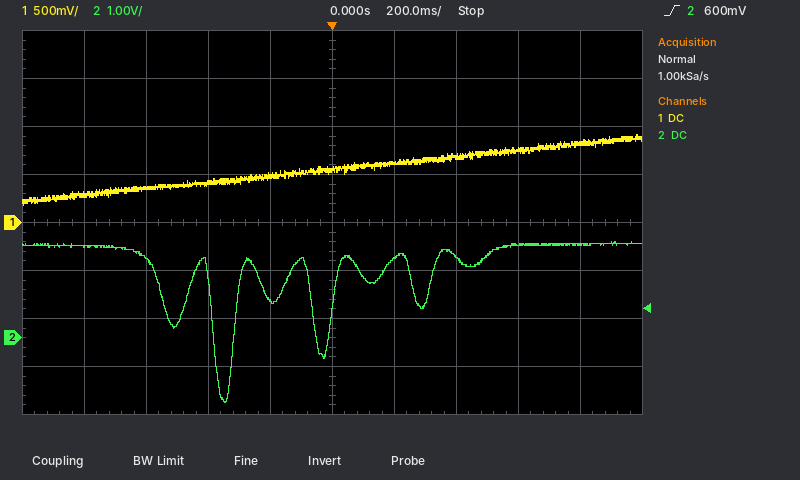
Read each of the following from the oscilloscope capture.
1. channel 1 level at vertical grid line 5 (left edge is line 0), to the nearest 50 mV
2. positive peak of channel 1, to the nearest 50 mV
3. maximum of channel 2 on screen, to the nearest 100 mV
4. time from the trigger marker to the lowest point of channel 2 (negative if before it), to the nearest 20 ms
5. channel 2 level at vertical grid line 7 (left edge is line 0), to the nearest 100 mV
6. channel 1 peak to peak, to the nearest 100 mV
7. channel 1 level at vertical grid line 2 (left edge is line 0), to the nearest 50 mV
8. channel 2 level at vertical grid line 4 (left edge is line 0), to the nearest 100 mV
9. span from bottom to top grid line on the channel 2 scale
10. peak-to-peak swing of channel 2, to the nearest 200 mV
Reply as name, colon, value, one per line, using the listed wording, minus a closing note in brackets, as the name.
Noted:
channel 1 level at vertical grid line 5 (left edge is line 0), to the nearest 50 mV: 550 mV
positive peak of channel 1, to the nearest 50 mV: 900 mV
maximum of channel 2 on screen, to the nearest 100 mV: 2.0 V
time from the trigger marker to the lowest point of channel 2 (negative if before it), to the nearest 20 ms: -340 ms
channel 2 level at vertical grid line 7 (left edge is line 0), to the nearest 100 mV: 1.7 V
channel 1 peak to peak, to the nearest 100 mV: 700 mV
channel 1 level at vertical grid line 2 (left edge is line 0), to the nearest 50 mV: 350 mV
channel 2 level at vertical grid line 4 (left edge is line 0), to the nearest 100 mV: 800 mV
span from bottom to top grid line on the channel 2 scale: 8 V
peak-to-peak swing of channel 2, to the nearest 200 mV: 3.4 V
